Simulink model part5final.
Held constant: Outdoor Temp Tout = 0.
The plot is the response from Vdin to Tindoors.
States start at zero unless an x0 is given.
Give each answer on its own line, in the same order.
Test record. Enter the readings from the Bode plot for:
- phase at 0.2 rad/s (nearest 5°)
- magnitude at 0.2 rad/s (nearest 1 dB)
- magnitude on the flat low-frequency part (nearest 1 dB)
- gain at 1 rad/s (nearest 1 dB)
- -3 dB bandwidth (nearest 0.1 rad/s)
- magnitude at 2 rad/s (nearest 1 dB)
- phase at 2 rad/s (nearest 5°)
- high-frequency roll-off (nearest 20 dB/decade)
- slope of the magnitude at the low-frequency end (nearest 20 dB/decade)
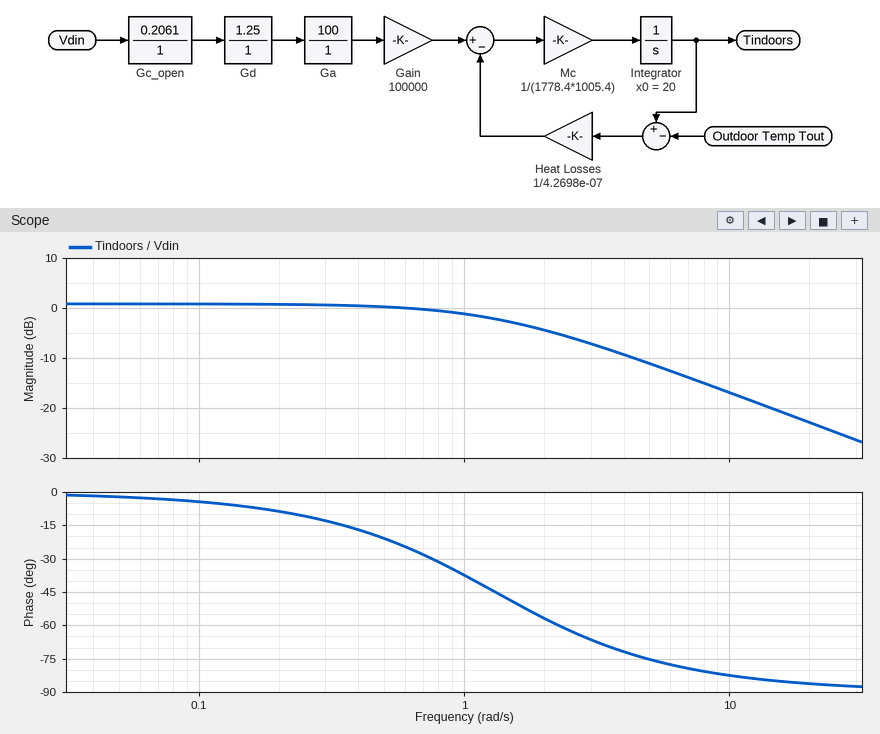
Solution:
-10°
1 dB
1 dB
-1 dB
1.3 rad/s
-4 dB
-55°
-20 dB/decade
0 dB/decade
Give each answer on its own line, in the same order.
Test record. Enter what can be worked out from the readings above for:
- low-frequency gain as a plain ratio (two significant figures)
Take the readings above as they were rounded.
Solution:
1.1
